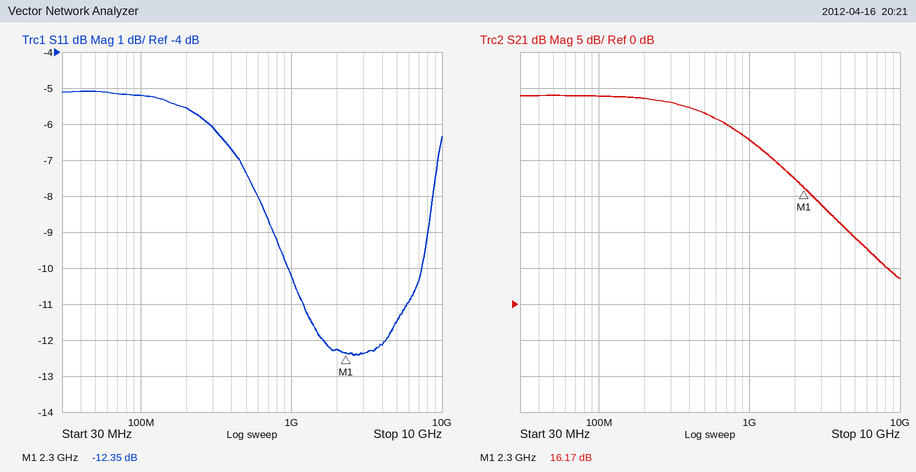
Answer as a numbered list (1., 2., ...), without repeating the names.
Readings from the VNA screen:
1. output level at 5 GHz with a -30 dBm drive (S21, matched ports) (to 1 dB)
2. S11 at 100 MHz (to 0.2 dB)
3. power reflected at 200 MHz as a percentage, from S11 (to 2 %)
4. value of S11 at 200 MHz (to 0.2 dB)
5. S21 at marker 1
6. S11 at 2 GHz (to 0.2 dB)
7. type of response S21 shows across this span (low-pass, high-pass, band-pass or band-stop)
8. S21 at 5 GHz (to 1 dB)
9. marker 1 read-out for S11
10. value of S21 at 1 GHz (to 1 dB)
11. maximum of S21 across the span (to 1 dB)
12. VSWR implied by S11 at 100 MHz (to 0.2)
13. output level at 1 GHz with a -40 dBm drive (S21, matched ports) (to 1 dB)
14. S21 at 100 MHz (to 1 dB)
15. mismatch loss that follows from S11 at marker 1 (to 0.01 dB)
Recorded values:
1. -21 dBm
2. -5.2 dB
3. 28 %
4. -5.6 dB
5. 16.17 dB
6. -12.2 dB
7. low-pass
8. 9 dB
9. -12.35 dB
10. 23 dB
11. 29 dB
12. 3.4
13. -17 dBm
14. 29 dB
15. 0.26 dB
